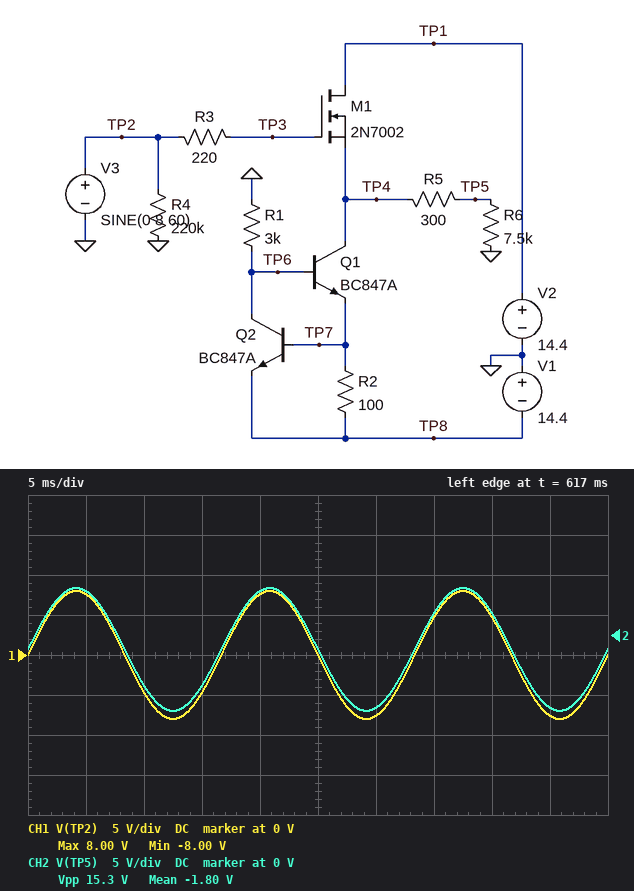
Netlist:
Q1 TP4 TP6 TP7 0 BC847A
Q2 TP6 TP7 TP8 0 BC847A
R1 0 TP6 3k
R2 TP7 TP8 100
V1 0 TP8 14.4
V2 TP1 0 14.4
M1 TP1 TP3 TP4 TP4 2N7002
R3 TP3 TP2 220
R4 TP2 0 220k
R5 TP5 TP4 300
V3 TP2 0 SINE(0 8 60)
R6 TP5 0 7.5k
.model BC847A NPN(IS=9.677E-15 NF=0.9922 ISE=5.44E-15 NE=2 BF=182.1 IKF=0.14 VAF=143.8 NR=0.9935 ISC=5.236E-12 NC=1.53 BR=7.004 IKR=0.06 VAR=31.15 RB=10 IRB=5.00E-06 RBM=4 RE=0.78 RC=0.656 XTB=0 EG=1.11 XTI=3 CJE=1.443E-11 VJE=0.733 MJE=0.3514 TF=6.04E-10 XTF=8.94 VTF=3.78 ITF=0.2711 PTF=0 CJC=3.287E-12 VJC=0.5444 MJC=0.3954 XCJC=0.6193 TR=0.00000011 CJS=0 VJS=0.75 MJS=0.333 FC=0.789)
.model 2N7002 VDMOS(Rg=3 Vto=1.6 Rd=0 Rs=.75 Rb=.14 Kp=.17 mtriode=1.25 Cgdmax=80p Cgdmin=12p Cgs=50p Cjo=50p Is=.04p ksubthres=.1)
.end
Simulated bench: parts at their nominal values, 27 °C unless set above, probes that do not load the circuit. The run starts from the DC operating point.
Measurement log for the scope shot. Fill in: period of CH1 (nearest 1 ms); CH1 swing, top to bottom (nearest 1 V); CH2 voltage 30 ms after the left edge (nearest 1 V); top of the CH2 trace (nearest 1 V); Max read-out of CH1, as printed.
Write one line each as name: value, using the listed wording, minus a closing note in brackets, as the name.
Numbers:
period of CH1: 17 ms
CH1 swing, top to bottom: 16 V
CH2 voltage 30 ms after the left edge: -9 V
top of the CH2 trace: 6 V
Max read-out of CH1, as printed: 8.00 V
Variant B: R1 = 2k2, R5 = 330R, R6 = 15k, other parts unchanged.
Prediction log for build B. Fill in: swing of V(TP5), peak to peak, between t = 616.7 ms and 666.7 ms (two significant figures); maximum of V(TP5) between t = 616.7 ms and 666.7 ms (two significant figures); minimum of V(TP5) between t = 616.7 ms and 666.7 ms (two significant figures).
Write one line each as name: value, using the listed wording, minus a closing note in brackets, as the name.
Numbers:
swing of V(TP5), peak to peak, between t = 616.7 ms and 666.7 ms: 16 V
maximum of V(TP5) between t = 616.7 ms and 666.7 ms: 6.0 V
minimum of V(TP5) between t = 616.7 ms and 666.7 ms: -9.7 V
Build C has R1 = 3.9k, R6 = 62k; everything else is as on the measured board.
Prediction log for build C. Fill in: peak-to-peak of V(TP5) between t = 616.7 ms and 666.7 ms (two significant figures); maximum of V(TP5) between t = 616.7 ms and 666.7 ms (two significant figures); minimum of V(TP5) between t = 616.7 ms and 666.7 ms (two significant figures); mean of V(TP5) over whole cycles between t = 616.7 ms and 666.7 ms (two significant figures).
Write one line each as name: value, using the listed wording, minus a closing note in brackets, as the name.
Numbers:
peak-to-peak of V(TP5) between t = 616.7 ms and 666.7 ms: 16 V
maximum of V(TP5) between t = 616.7 ms and 666.7 ms: 6.1 V
minimum of V(TP5) between t = 616.7 ms and 666.7 ms: -9.8 V
mean of V(TP5) over whole cycles between t = 616.7 ms and 666.7 ms: -1.9 V
